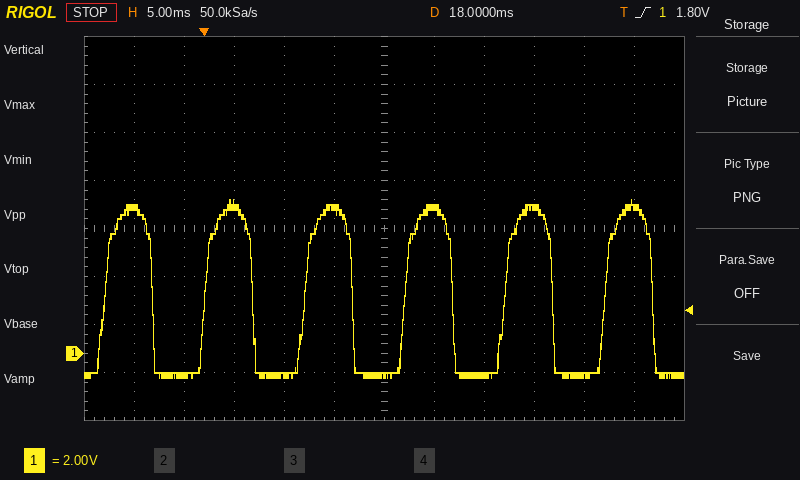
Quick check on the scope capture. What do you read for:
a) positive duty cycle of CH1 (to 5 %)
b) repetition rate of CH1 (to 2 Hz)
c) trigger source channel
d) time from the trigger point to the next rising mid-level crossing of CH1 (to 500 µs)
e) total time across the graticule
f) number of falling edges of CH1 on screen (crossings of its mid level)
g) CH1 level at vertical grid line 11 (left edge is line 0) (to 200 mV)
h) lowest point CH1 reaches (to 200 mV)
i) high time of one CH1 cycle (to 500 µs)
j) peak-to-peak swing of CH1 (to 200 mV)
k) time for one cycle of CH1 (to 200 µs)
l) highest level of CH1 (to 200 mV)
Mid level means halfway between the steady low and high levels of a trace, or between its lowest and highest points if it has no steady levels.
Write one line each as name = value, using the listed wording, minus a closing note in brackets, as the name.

positive duty cycle of CH1 = 45 %
repetition rate of CH1 = 100 Hz
trigger source channel = CH1
time from the trigger point to the next rising mid-level crossing of CH1 = 10.0 ms
total time across the graticule = 60 ms
number of falling edges of CH1 on screen = 6
CH1 level at vertical grid line 11 (left edge is line 0) = 6.2 V
lowest point CH1 reaches = -1.0 V
high time of one CH1 cycle = 4.5 ms
peak-to-peak swing of CH1 = 7.4 V
time for one cycle of CH1 = 10.0 ms
highest level of CH1 = 6.4 V
